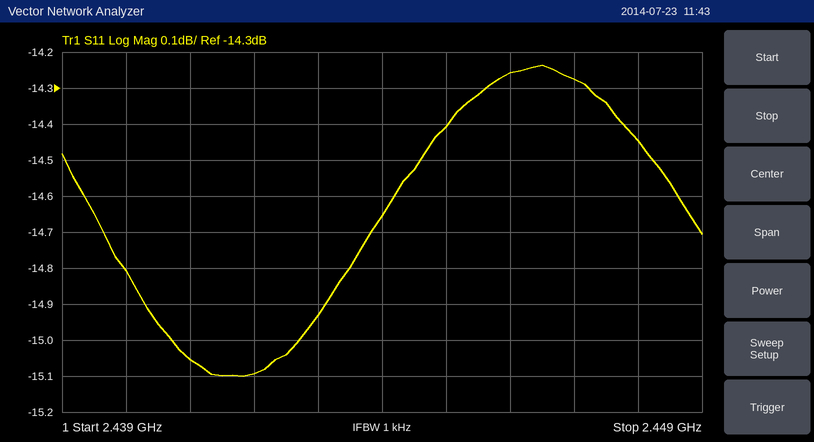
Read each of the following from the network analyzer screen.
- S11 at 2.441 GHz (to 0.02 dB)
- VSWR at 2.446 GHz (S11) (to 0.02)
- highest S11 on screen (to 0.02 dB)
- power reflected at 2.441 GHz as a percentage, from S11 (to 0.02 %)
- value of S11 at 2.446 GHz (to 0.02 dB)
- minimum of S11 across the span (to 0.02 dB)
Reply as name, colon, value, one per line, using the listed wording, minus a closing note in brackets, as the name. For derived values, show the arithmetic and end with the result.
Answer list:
S11 at 2.441 GHz: -15.06 dB
VSWR at 2.446 GHz (S11): |Γ| = 10^(-14.26/20) = 0.1936; VSWR = (1 + 0.1936)/(1 − 0.1936) ≈ 1.48
highest S11 on screen: -14.24 dB
power reflected at 2.441 GHz as a percentage, from S11: 10^(-15.06/10) ≈ 3.12 %
value of S11 at 2.446 GHz: -14.26 dB
minimum of S11 across the span: -15.10 dB
